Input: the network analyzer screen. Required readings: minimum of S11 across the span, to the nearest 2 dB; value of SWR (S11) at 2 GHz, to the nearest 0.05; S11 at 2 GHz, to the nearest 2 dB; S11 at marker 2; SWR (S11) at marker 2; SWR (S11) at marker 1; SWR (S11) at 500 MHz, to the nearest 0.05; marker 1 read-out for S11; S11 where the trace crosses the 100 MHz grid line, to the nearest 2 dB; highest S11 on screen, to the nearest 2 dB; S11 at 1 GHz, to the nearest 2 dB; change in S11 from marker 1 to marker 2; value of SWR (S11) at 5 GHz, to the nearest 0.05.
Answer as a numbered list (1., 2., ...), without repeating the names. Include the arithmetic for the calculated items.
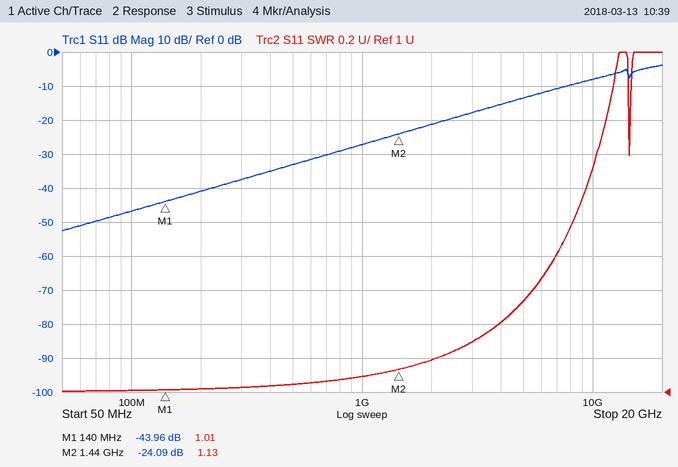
1. -52 dB
2. 1.20
3. -22 dB
4. -24.09 dB
5. 1.13
6. 1.01
7. 1.05
8. -43.96 dB
9. -46 dB
10. -4 dB
11. -28 dB
12. -24.09 − (-43.96) = 19.87 dB
13. 1.55
